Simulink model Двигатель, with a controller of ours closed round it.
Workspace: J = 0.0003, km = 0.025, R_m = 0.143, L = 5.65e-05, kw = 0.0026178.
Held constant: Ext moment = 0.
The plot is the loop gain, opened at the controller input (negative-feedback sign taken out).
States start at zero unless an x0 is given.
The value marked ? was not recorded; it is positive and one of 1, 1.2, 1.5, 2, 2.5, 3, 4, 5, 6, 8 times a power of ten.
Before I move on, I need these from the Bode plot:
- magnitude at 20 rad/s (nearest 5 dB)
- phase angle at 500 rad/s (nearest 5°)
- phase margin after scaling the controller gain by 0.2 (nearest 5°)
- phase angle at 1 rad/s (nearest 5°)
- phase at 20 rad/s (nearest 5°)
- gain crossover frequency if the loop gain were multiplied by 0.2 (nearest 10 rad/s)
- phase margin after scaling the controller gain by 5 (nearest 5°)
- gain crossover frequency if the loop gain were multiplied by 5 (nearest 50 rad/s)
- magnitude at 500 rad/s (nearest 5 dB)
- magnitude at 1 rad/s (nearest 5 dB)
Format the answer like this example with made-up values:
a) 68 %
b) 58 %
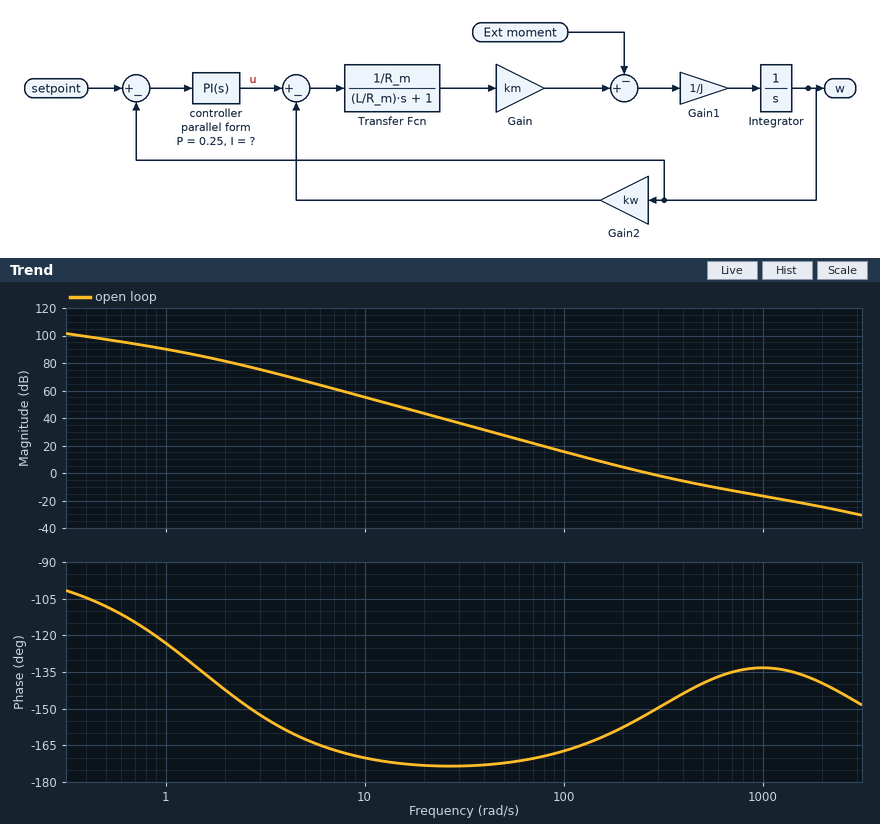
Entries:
a) 45 dB
b) -140°
c) 15°
d) -125°
e) -175°
f) 110 rad/s
g) 45°
h) 800 rad/s
i) -10 dB
j) 90 dB
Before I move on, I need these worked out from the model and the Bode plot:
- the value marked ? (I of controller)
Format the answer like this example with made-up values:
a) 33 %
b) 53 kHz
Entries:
a) 100
